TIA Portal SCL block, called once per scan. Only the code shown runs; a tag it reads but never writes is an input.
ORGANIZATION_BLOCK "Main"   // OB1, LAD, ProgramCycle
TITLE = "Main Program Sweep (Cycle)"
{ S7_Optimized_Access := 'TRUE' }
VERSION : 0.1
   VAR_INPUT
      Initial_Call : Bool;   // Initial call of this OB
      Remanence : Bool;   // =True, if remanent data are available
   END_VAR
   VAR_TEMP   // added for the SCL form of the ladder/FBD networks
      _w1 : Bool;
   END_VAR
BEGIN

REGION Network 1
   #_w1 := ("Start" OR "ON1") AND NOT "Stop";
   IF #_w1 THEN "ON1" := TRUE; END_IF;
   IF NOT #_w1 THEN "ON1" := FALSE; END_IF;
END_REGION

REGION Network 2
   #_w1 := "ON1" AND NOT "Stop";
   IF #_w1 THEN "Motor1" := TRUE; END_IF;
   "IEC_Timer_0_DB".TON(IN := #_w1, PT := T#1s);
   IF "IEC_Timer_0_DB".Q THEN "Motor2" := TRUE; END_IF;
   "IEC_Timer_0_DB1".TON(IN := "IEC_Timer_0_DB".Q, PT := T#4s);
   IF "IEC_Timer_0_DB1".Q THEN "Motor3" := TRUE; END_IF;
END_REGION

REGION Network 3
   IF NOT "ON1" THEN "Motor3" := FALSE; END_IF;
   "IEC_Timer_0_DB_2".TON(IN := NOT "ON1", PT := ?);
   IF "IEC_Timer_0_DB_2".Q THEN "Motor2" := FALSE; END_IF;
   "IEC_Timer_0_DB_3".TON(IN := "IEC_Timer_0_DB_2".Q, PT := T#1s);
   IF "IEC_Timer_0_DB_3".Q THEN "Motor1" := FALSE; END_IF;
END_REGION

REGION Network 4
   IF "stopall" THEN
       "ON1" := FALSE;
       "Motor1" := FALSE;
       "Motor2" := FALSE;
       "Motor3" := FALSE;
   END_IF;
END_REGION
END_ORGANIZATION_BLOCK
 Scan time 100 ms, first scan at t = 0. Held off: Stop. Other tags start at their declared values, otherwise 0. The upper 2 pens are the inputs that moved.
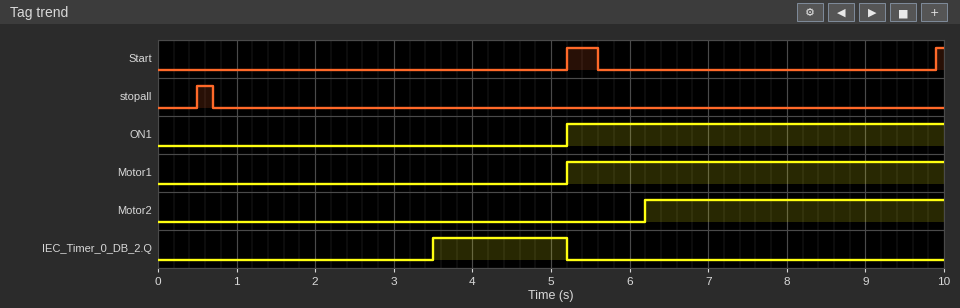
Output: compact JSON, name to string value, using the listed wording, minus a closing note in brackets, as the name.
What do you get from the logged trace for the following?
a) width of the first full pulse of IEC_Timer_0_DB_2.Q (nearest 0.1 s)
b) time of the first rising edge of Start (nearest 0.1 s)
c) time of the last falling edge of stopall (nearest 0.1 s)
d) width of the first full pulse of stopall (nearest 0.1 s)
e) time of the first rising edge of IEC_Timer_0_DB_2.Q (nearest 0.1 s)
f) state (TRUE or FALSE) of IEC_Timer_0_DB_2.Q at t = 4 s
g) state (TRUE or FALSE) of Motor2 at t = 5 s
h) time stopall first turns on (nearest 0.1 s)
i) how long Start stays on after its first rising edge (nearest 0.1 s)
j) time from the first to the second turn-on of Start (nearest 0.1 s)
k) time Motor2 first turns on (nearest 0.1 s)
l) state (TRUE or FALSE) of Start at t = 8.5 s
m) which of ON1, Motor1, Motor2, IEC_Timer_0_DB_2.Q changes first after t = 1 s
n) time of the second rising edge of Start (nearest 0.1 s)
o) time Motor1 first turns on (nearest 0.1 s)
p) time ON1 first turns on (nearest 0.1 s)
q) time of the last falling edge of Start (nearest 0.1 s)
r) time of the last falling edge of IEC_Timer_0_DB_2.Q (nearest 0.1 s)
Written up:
{"width of the first full pulse of IEC_Timer_0_DB_2.Q": "1.7 s", "time of the first rising edge of Start": "5.2 s", "time of the last falling edge of stopall": "0.7 s", "width of the first full pulse of stopall": "0.2 s", "time of the first rising edge of IEC_Timer_0_DB_2.Q": "3.5 s", "state (TRUE or FALSE) of IEC_Timer_0_DB_2.Q at t = 4 s": "TRUE", "state (TRUE or FALSE) of Motor2 at t = 5 s": "FALSE", "time stopall first turns on": "0.5 s", "how long Start stays on after its first rising edge": "0.4 s", "time from the first to the second turn-on of Start": "4.7 s", "time Motor2 first turns on": "6.2 s", "state (TRUE or FALSE) of Start at t = 8.5 s": "FALSE", "which of ON1, Motor1, Motor2, IEC_Timer_0_DB_2.Q changes first after t = 1 s": "IEC_Timer_0_DB_2.Q", "time of the second rising edge of Start": "9.9 s", "time Motor1 first turns on": "5.2 s", "time ON1 first turns on": "5.2 s", "time of the last falling edge of Start": "5.6 s", "time of the last falling edge of IEC_Timer_0_DB_2.Q": "5.2 s"}
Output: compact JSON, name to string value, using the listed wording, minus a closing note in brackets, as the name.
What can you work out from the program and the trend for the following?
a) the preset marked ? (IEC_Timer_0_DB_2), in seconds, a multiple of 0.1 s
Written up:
{"the preset marked ? (IEC_Timer_0_DB_2), in seconds, a multiple of 0.1 s": "3.5 s"}
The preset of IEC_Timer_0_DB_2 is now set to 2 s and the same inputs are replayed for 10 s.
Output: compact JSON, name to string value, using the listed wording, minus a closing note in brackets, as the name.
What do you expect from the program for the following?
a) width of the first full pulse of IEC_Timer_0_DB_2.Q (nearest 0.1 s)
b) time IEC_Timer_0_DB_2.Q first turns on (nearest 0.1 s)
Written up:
{"width of the first full pulse of IEC_Timer_0_DB_2.Q": "3.2 s", "time IEC_Timer_0_DB_2.Q first turns on": "2.0 s"}
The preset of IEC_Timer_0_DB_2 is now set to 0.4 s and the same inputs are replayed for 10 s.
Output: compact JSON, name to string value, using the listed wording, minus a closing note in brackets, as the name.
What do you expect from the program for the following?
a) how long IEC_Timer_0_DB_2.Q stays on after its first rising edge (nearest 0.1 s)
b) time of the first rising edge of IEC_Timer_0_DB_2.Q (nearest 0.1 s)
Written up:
{"how long IEC_Timer_0_DB_2.Q stays on after its first rising edge": "4.8 s", "time of the first rising edge of IEC_Timer_0_DB_2.Q": "0.4 s"}
